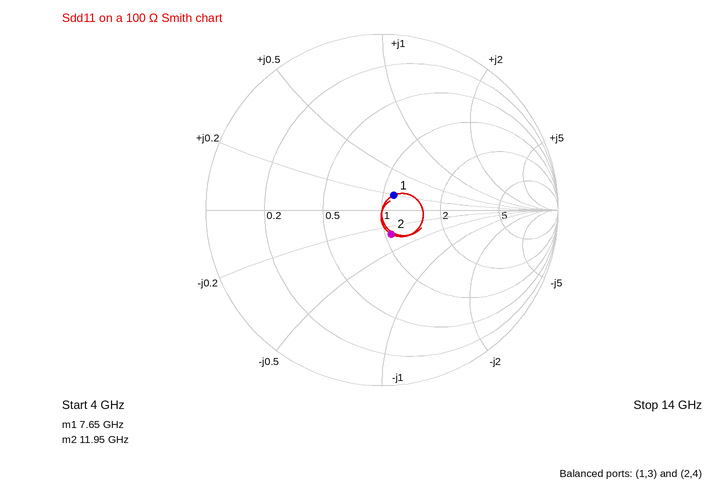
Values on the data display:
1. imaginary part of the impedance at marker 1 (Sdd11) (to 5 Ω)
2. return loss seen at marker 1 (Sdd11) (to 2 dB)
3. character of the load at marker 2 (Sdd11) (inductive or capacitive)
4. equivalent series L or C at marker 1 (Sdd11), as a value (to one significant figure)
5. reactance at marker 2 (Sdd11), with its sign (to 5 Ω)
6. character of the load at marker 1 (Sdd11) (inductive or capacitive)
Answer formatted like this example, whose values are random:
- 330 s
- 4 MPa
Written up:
- +20 Ω
- 20 dB
- capacitive
- 400 pH
- -30 Ω
- inductive
